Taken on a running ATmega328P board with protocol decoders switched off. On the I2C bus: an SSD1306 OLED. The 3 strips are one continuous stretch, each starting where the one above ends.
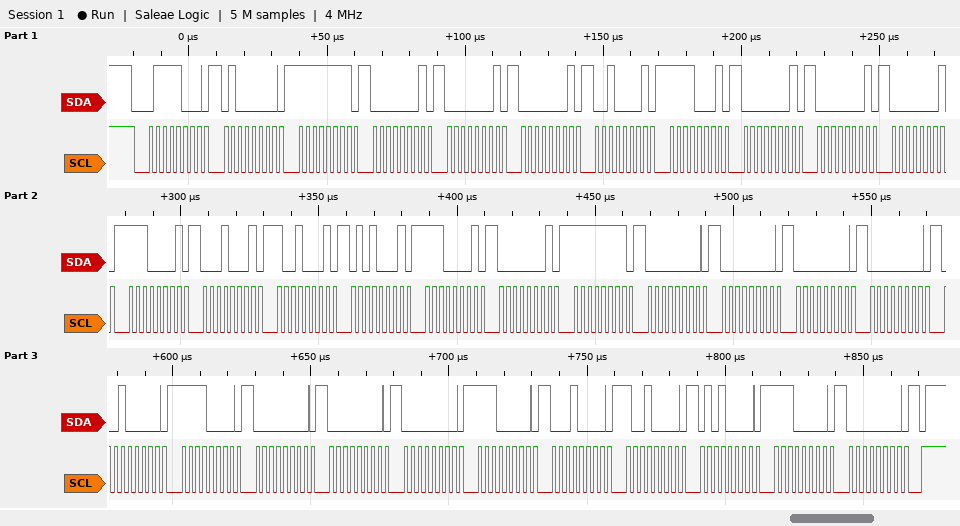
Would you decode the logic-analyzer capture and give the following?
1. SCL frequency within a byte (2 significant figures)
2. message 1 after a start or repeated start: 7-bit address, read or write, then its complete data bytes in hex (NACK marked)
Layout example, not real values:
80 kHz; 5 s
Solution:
400 kHz; 0x3C write: 40 FF 01 01 01 21 F1 01 01 01 E1 11 91 51 E1 01 FF 00 00 00 00 20 F0 00 00 00 E0 10 90 50 E0 00
